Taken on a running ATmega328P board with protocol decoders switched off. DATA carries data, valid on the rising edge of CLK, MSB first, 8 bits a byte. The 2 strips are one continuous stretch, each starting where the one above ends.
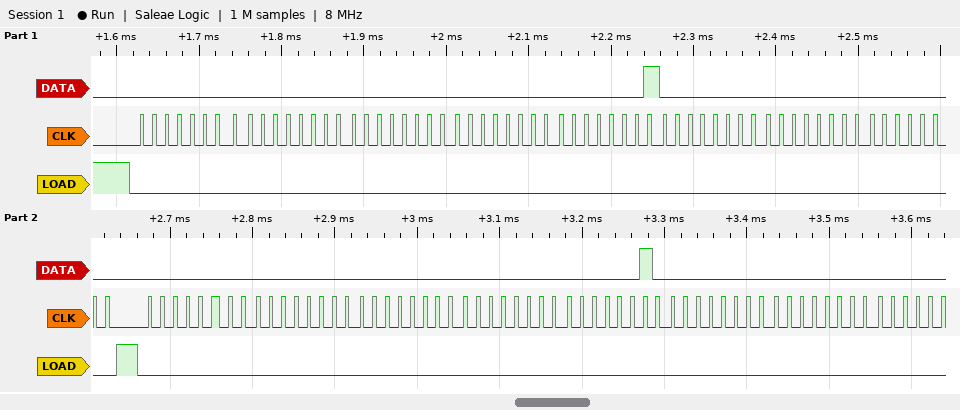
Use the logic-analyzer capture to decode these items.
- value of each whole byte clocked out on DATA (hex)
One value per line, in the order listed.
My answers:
00 00 00 00 01 00 00 00 00 00 00 00 02 00 00
